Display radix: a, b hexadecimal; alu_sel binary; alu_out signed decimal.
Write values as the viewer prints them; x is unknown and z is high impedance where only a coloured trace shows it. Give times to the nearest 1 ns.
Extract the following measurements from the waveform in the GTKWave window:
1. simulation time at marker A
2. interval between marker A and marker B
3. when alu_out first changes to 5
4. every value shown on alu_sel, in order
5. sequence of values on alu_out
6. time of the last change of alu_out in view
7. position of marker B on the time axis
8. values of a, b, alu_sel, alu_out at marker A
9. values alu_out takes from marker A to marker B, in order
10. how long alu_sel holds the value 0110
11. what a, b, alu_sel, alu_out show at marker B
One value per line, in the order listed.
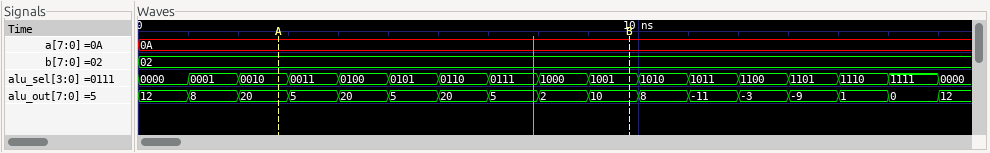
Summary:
3 ns
7 ns
3 ns
0000, 0001, 0010, 0011, 0100, 0101, 0110, 0111, 1000, 1001, 1010, 1011, 1100, 1101, 1110, 1111, 0000
12, 8, 20, 5, 20, 5, 20, 5, 2, 10, 8, -11, -3, -9, 1, 0, 12
16 ns
10 ns
a=0A, b=02, alu_sel=0010, alu_out=20
20, 5, 20, 5, 20, 5, 2, 10
1 ns
a=0A, b=02, alu_sel=1001, alu_out=10
